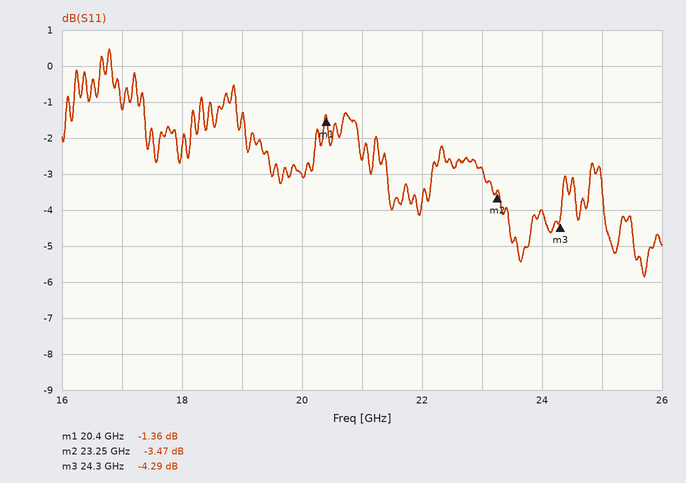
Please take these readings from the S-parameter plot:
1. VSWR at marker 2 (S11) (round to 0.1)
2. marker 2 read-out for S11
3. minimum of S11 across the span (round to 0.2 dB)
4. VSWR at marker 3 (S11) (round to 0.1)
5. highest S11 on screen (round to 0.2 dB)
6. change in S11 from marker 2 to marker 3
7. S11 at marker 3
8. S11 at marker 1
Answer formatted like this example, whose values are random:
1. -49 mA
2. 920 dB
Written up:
1. 5.1
2. -3.47 dB
3. -5.8 dB
4. 4.1
5. 0.4 dB
6. -0.82 dB
7. -4.29 dB
8. -1.36 dB
